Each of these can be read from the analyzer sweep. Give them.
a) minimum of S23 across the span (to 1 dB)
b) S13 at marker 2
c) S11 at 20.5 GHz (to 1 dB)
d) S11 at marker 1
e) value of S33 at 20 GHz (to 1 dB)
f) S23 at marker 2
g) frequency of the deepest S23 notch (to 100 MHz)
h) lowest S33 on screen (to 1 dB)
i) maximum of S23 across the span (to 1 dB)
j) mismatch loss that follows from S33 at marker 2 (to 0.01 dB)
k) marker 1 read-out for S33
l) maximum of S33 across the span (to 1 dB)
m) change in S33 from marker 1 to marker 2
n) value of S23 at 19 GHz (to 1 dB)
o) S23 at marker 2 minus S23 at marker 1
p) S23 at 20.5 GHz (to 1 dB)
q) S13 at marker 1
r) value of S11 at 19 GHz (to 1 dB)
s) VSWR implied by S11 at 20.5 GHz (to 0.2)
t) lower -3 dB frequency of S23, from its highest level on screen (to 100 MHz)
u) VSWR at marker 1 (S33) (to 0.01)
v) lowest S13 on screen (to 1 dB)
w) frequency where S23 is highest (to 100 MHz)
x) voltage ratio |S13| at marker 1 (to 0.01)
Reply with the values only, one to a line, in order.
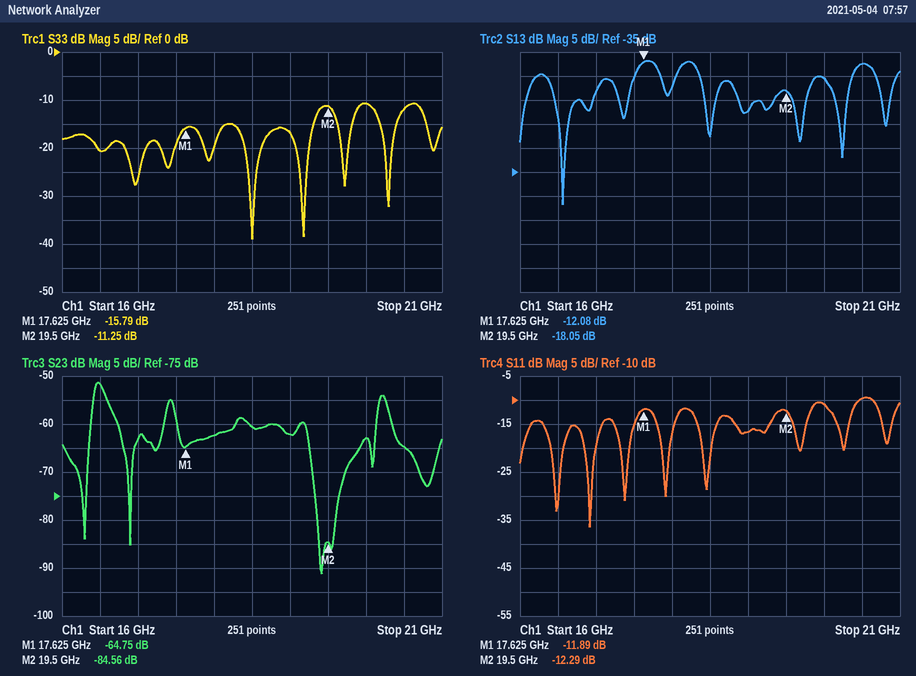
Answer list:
-91 dB
-18.05 dB
-10 dB
-11.89 dB
-11 dB
-84.56 dB
19.4 GHz
-39 dB
-51 dB
0.34 dB
-15.79 dB
-11 dB
4.54 dB
-62 dB
-19.81 dB
-65 dB
-12.08 dB
-17 dB
2.0
16.4 GHz
1.39
-42 dB
16.5 GHz
0.25
